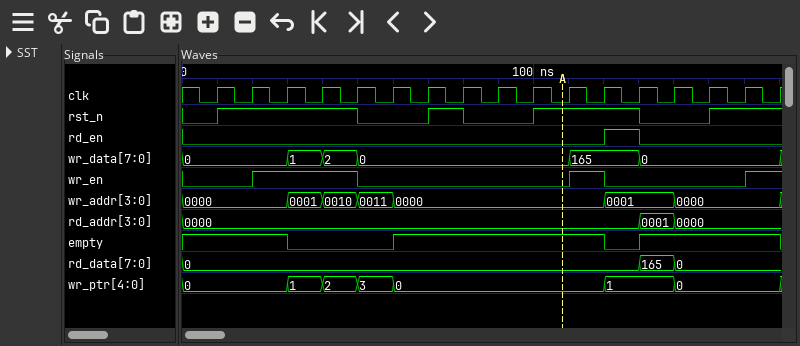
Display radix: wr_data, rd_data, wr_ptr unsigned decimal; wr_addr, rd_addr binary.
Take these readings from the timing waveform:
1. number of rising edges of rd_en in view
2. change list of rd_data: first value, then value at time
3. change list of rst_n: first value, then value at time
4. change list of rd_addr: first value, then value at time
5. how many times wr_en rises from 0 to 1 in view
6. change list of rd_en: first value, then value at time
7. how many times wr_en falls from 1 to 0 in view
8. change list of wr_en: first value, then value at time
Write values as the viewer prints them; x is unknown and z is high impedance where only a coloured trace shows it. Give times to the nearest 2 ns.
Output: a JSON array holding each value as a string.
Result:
["1", "0, 165 at 130 ns, 0 at 140 ns", "0, 1 at 10 ns, 0 at 50 ns, 1 at 70 ns, 0 at 80 ns, 1 at 100 ns, 0 at 130 ns, 1 at 150 ns", "0000, 0001 at 130 ns, 0000 at 140 ns", "3", "0, 1 at 120 ns, 0 at 130 ns", "2", "0, 1 at 20 ns, 0 at 50 ns, 1 at 110 ns, 0 at 120 ns, 1 at 160 ns"]
